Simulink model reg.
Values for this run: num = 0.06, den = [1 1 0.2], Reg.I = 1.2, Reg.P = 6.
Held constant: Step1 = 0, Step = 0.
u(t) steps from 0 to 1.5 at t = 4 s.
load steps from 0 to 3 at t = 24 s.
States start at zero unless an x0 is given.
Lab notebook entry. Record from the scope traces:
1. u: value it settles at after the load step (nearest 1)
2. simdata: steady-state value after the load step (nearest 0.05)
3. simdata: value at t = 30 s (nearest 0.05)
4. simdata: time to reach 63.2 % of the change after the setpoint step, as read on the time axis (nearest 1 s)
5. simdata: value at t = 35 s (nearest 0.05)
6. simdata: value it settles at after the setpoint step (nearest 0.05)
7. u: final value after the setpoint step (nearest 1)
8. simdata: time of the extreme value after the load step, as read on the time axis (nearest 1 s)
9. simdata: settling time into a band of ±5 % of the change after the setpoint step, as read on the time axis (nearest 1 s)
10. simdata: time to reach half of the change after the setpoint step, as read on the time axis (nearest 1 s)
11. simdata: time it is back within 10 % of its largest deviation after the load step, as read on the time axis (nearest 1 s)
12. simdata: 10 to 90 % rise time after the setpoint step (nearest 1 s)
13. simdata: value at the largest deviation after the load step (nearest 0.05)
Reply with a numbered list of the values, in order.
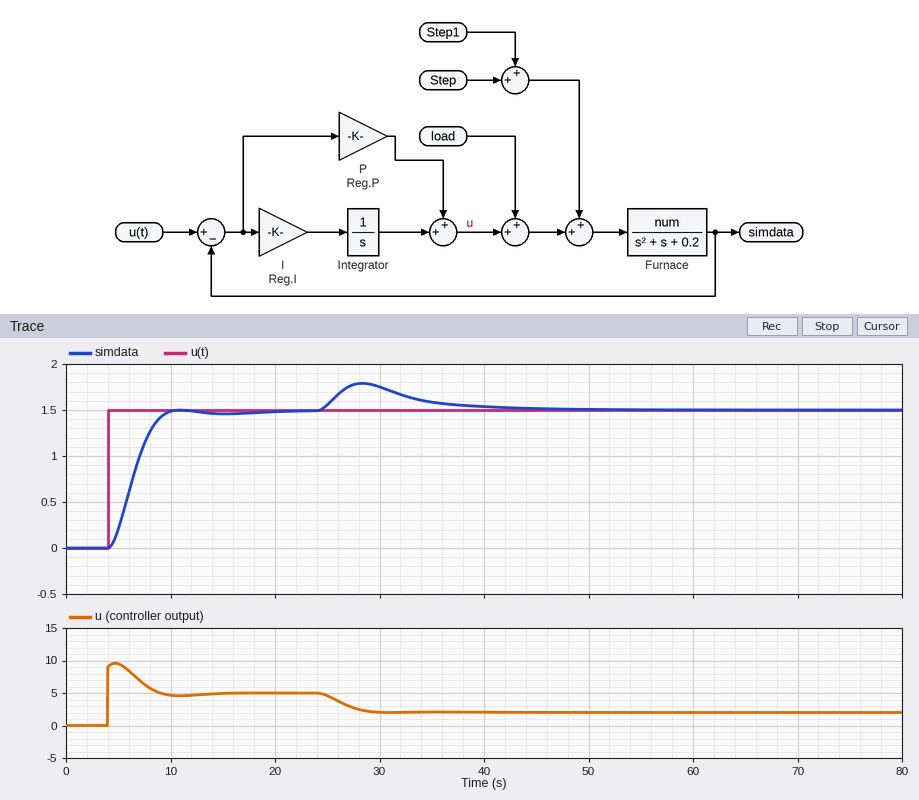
1. 2
2. 1.50
3. 1.75
4. 7 s
5. 1.60
6. 1.50
7. 5
8. 28 s
9. 9 s
10. 6 s
11. 41 s
12. 4 s
13. 1.80
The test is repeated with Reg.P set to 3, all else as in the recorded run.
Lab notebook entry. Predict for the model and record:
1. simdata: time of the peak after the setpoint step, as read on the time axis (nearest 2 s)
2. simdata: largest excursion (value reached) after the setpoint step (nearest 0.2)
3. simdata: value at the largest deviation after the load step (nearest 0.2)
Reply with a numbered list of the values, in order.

1. 14 s
2. 1.6
3. 1.8
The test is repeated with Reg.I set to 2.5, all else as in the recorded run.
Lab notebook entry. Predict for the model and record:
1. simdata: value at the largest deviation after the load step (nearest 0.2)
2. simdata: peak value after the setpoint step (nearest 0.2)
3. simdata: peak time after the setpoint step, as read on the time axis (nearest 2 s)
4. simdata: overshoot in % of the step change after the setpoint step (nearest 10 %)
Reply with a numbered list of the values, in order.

1. 1.8
2. 1.8
3. 10 s
4. 20 %
